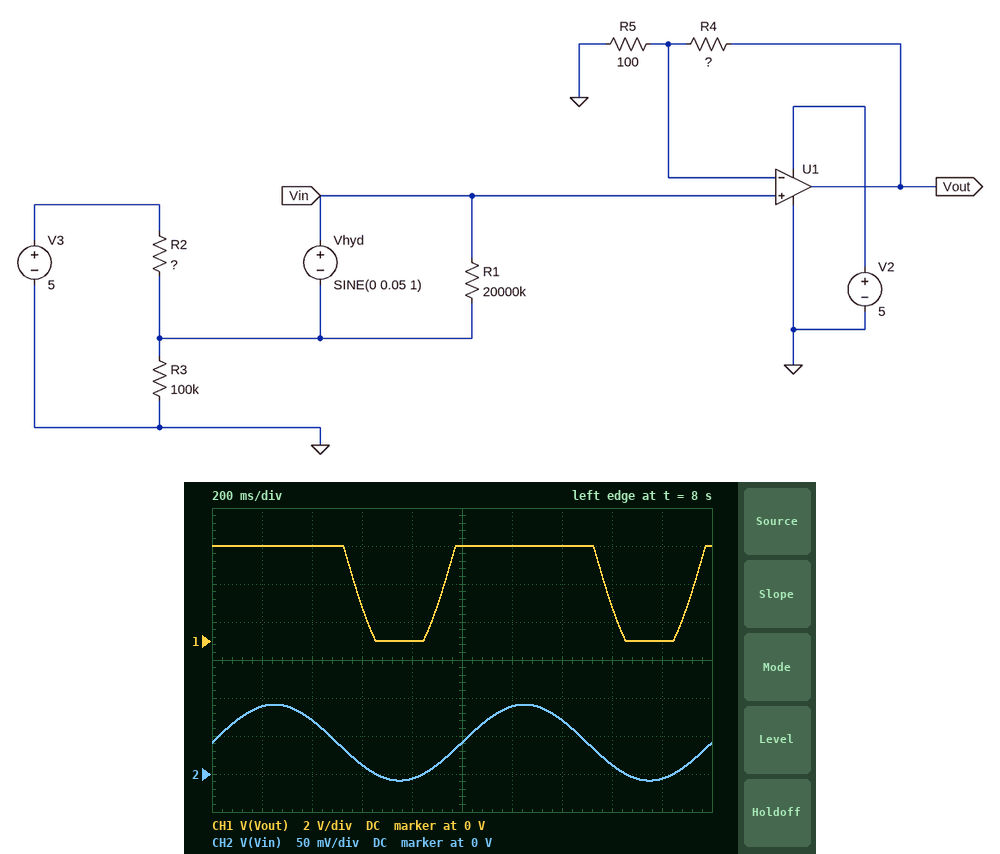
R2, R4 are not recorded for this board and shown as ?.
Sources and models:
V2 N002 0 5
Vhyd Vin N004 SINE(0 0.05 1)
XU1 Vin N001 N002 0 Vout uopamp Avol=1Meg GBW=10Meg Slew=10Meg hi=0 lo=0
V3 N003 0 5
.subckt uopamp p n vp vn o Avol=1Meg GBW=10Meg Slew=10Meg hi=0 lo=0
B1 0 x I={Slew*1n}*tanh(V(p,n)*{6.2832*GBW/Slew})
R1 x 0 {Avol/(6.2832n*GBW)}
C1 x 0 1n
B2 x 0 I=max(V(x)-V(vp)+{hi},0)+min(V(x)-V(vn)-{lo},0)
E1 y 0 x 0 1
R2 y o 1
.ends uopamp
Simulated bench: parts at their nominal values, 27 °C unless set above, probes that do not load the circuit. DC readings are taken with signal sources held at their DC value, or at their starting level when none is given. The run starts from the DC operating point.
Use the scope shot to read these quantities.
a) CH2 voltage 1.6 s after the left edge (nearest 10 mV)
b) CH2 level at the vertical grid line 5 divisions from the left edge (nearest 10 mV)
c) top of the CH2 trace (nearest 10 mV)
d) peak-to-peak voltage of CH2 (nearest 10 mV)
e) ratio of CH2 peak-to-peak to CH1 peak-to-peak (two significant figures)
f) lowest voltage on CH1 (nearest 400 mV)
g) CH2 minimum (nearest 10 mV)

10 mV
40 mV
90 mV
100 mV
0.020
0 V
-10 mV
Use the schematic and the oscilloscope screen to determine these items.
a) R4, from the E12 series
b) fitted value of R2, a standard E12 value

15 kΩ
12 MΩ
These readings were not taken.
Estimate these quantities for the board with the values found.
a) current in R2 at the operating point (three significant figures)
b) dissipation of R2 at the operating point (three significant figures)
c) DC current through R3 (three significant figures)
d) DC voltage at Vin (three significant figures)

413 nA
2.05 µW
413 nA
41.3 mV
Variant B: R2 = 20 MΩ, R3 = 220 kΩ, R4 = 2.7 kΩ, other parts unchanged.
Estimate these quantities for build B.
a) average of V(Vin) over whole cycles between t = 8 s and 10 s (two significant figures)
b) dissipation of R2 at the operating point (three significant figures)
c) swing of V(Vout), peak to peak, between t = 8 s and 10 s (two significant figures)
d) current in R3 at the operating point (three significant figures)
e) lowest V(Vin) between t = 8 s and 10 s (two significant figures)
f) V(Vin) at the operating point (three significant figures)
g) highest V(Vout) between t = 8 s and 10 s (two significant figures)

54 mV
1.22 µW
2.8 V
247 nA
4.4 mV
54.4 mV
2.9 V
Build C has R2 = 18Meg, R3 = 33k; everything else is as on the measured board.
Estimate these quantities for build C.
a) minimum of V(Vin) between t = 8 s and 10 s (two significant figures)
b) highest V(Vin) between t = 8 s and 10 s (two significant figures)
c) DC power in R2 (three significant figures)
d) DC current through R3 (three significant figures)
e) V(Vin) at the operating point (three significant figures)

-41 mV
59 mV
1.38 µW
277 nA
9.15 mV
